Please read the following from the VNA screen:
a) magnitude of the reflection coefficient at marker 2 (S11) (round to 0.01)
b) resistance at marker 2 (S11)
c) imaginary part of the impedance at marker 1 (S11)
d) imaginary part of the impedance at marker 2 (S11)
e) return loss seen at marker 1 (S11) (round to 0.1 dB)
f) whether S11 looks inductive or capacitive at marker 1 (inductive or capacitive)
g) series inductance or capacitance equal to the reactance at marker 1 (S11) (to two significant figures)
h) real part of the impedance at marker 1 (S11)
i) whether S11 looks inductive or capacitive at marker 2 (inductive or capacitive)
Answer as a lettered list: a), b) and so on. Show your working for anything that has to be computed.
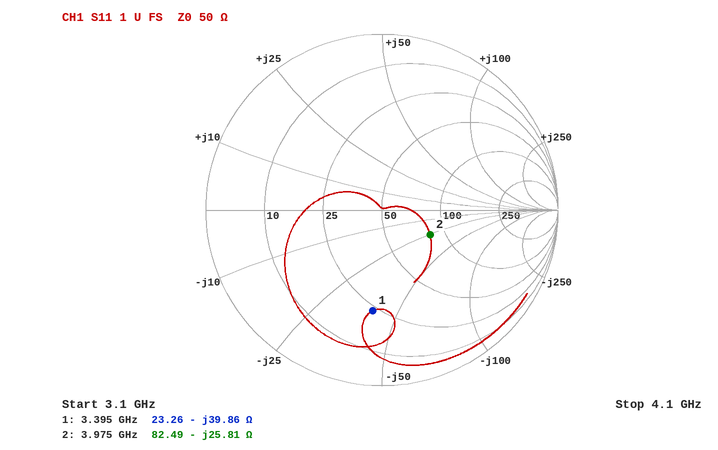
a) 0.31
b) 82.49 Ω
c) -39.86 Ω
d) -25.81 Ω
e) 4.8 dB
f) capacitive
g) C = 1/(2π × 3.395 GHz × 39.86 Ω) ≈ 1.2 pF
h) 23.26 Ω
i) capacitive
